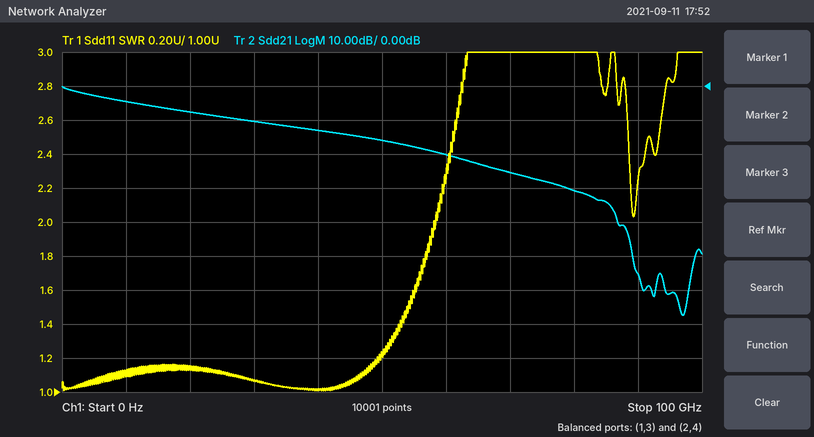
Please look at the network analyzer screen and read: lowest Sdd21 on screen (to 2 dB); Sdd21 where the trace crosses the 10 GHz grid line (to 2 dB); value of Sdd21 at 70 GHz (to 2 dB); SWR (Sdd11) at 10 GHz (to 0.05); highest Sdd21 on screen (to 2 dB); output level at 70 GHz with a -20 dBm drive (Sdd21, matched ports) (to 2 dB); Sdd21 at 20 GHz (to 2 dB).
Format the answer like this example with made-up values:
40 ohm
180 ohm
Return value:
-68 dB
-4 dB
-26 dB
1.10
0 dB
-46 dBm
-8 dB
